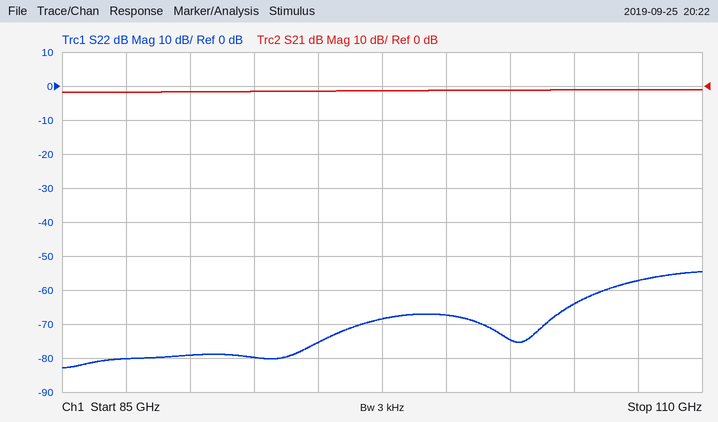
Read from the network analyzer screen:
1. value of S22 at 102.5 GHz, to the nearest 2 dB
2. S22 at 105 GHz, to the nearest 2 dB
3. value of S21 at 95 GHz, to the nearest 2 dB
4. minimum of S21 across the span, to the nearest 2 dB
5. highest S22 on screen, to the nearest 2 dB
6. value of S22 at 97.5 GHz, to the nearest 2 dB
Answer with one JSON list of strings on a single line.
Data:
["-74 dB", "-64 dB", "-2 dB", "-2 dB", "-54 dB", "-68 dB"]
